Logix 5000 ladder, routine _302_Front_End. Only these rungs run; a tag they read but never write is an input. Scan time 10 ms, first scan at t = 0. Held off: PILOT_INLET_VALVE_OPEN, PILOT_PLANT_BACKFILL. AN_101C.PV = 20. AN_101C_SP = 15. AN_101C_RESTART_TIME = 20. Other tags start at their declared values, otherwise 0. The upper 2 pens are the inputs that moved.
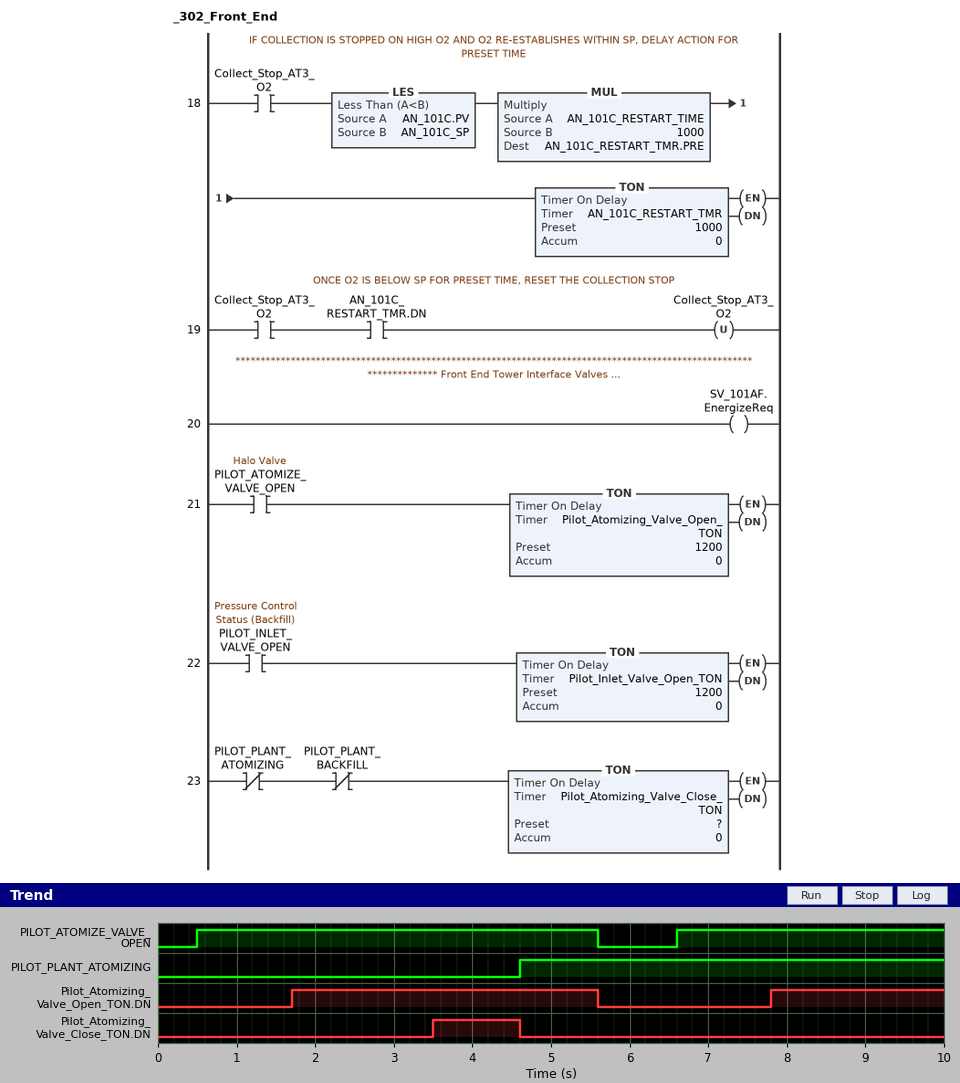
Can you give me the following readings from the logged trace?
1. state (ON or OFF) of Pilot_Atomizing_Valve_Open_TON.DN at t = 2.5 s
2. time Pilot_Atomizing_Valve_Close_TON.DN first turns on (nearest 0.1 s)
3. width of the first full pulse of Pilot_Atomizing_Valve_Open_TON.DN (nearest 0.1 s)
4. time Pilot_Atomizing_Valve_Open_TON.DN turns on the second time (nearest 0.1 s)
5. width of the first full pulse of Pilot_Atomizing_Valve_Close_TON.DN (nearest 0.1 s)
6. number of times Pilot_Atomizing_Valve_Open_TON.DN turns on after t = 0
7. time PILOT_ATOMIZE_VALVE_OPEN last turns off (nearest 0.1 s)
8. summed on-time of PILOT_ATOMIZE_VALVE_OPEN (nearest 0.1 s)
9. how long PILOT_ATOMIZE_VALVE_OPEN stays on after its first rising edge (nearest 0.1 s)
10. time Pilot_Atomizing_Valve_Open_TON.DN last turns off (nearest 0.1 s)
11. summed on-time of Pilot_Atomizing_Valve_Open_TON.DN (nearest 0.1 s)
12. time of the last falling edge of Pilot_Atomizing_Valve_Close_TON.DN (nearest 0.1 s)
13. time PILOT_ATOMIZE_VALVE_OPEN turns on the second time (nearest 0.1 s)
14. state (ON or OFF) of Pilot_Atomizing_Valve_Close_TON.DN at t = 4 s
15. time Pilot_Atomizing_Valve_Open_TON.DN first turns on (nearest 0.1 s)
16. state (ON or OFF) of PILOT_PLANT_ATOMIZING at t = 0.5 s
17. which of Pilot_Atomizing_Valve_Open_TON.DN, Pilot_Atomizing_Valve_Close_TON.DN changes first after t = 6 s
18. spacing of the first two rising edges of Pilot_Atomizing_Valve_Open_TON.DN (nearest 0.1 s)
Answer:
ON
3.5 s
3.9 s
7.8 s
1.1 s
2
5.6 s
8.5 s
5.1 s
5.6 s
6.1 s
4.6 s
6.6 s
ON
1.7 s
OFF
Pilot_Atomizing_Valve_Open_TON.DN
6.1 s
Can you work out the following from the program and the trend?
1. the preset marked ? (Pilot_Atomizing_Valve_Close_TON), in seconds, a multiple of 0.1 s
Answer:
3.5 s
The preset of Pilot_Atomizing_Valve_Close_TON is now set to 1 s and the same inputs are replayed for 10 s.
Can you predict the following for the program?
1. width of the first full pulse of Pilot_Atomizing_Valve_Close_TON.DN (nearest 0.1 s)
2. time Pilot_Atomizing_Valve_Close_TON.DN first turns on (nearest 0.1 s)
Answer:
3.6 s
1.0 s
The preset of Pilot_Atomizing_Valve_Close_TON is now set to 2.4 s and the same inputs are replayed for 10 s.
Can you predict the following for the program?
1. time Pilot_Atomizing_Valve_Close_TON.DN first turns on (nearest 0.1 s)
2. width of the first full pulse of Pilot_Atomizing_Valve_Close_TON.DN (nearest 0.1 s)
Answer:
2.4 s
2.2 s
